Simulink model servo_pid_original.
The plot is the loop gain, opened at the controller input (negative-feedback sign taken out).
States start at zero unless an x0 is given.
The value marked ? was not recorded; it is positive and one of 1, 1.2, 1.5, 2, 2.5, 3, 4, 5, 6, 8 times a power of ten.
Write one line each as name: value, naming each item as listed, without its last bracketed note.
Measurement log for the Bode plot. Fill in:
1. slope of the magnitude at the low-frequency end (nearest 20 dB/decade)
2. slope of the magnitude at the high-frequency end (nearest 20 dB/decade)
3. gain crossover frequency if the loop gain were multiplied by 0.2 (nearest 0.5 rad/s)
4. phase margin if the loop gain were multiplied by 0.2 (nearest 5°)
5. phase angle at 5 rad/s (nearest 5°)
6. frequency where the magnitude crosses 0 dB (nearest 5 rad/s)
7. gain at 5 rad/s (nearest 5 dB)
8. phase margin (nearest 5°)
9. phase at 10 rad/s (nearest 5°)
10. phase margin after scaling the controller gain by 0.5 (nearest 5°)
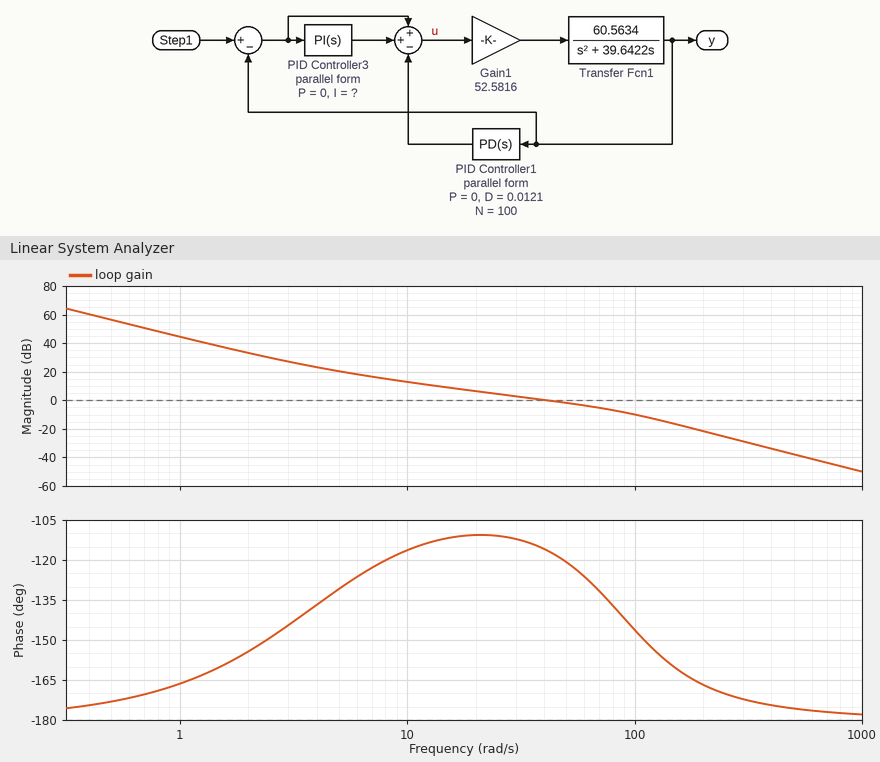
slope of the magnitude at the low-frequency end: -40 dB/decade
slope of the magnitude at the high-frequency end: -40 dB/decade
gain crossover frequency if the loop gain were multiplied by 0.2: 9.0 rad/s
phase margin if the loop gain were multiplied by 0.2: 60°
phase angle at 5 rad/s: -130°
frequency where the magnitude crosses 0 dB: 40 rad/s
gain at 5 rad/s: 20 dB
phase margin: 65°
phase at 10 rad/s: -115°
phase margin after scaling the controller gain by 0.5: 70°
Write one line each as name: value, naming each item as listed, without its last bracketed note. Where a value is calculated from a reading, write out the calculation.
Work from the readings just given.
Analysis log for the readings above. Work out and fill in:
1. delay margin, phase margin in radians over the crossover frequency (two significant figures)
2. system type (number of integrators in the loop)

delay margin, phase margin in radians over the crossover frequency: 65 × π / 180 / 40 = 0.028 s
system type: 2
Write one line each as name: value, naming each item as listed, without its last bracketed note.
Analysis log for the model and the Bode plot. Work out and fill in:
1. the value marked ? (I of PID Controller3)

the value marked ?: 4
